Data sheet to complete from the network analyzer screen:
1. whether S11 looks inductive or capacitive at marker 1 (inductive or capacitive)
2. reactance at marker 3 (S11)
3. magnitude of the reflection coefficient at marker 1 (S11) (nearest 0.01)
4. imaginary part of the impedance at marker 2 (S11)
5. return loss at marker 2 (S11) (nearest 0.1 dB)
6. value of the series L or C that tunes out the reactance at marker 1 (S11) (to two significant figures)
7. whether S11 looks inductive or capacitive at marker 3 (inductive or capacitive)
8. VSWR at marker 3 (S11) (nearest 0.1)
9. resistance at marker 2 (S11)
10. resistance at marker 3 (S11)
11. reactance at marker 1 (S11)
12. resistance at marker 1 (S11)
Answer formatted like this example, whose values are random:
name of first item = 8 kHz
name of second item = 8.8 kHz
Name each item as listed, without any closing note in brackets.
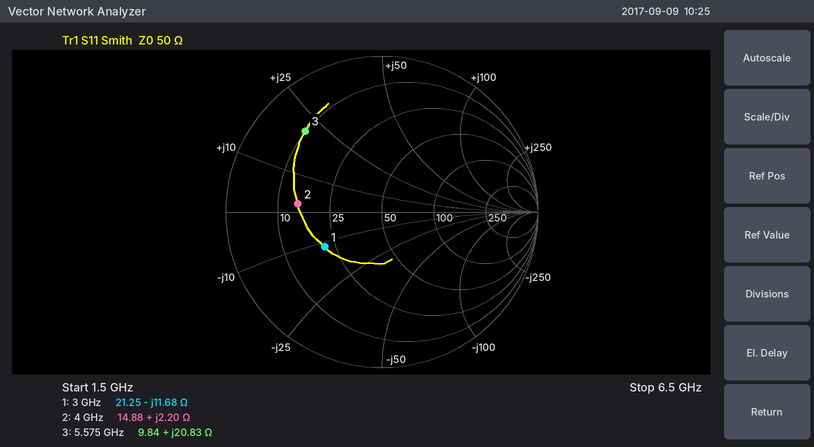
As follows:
whether S11 looks inductive or capacitive at marker 1 = capacitive
reactance at marker 3 = +20.83 Ω
magnitude of the reflection coefficient at marker 1 (S11) = 0.43
imaginary part of the impedance at marker 2 = +2.20 Ω
return loss at marker 2 (S11) = 5.3 dB
value of the series L or C that tunes out the reactance at marker 1 (S11) = 620 pH
whether S11 looks inductive or capacitive at marker 3 = inductive
VSWR at marker 3 (S11) = 6.0
resistance at marker 2 = 14.88 Ω
resistance at marker 3 = 9.84 Ω
reactance at marker 1 = -11.68 Ω
resistance at marker 1 = 21.25 Ω
